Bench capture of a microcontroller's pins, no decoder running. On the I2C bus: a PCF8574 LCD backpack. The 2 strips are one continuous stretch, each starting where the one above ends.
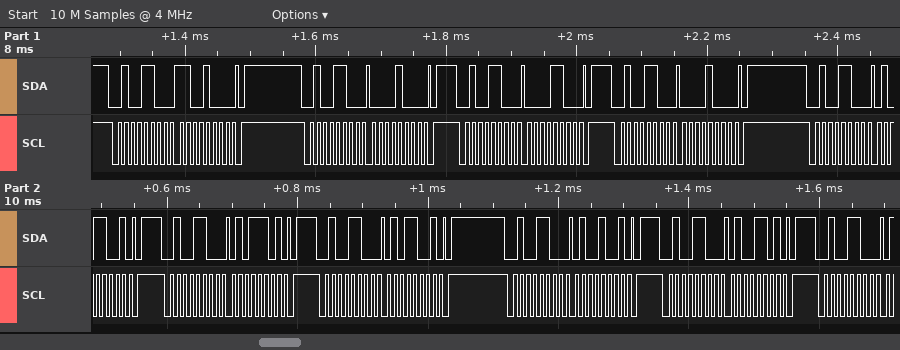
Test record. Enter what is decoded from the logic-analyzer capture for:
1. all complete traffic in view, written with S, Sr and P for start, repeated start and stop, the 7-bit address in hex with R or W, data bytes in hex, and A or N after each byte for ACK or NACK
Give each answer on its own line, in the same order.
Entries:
S 26W A C8 A P S 26W A 08 A P S 26W A 0C A P S 26W A 08 A P S 26W A 59 A P S 26W A 5D A P S 26W A 59 A P S 26W A 49 A P S 26W A 4D A P S 26W A
